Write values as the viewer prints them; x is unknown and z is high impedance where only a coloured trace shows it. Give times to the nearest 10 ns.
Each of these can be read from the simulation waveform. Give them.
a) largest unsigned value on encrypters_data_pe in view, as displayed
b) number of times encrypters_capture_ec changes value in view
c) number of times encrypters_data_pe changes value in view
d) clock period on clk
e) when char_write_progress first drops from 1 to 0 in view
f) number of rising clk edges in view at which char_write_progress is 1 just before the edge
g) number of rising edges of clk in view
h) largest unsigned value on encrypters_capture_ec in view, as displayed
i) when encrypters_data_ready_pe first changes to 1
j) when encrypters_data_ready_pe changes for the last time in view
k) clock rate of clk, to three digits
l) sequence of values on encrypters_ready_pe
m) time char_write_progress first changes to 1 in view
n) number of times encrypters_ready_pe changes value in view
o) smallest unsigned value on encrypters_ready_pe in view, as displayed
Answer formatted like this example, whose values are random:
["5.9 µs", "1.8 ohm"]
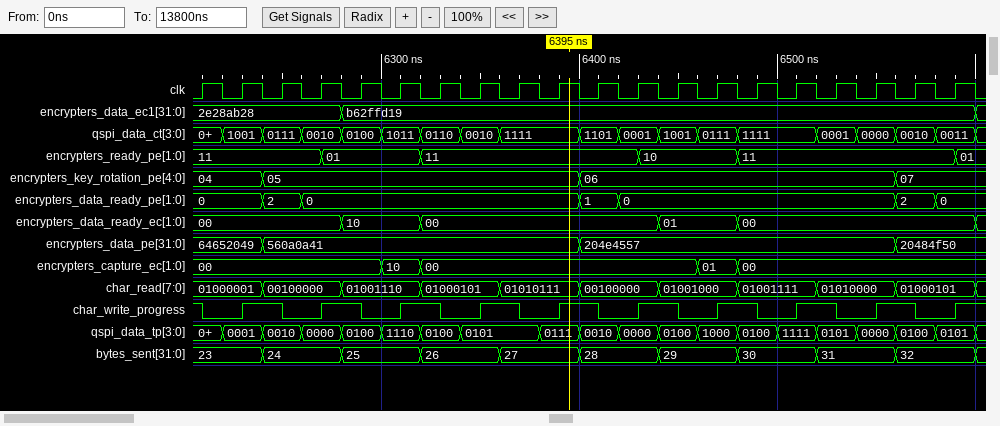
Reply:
["64652049", "4", "3", "20 ns", "6210 ns", "10", "20", "10", "6400 ns", "6580 ns", "50.0 MHz", "11, 01, 11, 10, 11, 01", "6230 ns", "5", "01"]
